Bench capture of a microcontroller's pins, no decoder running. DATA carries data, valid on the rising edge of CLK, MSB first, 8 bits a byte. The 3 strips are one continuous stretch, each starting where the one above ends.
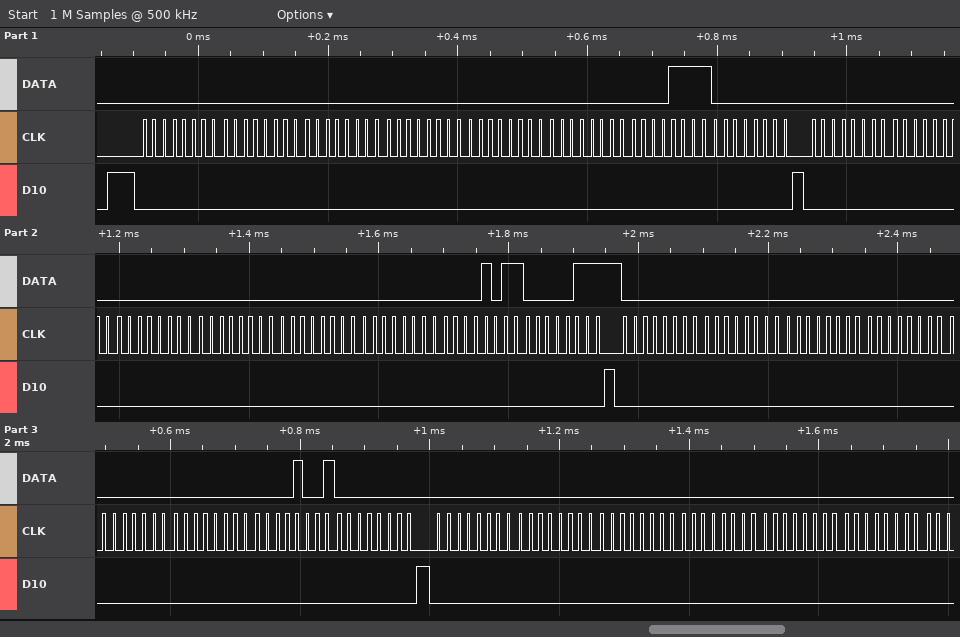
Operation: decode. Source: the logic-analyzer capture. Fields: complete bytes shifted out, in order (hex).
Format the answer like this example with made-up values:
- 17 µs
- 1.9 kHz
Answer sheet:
- 00 00 00 00 00 00 0F 00 00 00 00 00 00 00 0B 07 00 00 00 00 00 00 09 00 00 00 00 00 00 00
